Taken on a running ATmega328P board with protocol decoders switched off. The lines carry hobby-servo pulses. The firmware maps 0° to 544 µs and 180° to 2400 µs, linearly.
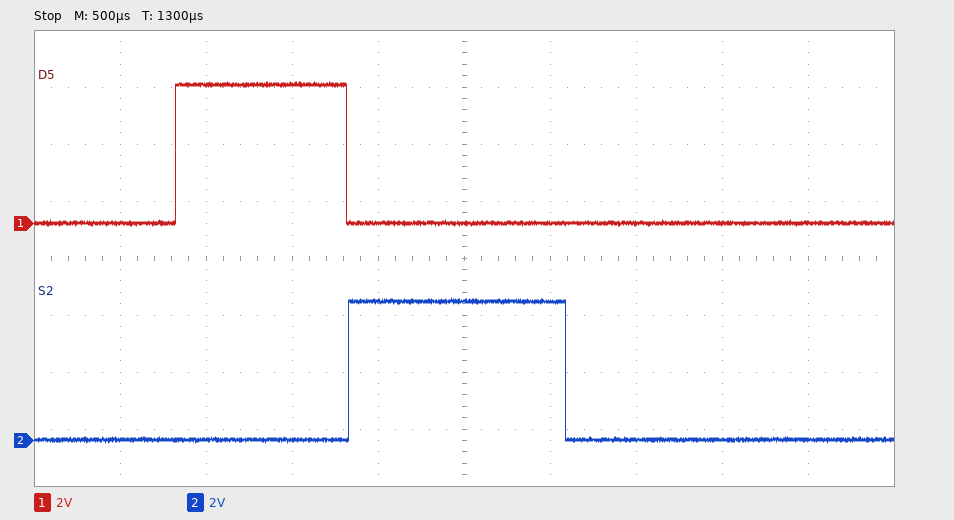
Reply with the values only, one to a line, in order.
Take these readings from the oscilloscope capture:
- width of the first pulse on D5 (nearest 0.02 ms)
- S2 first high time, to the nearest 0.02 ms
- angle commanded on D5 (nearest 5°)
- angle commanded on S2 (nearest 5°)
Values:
1.00 ms
1.26 ms
45°
70°
